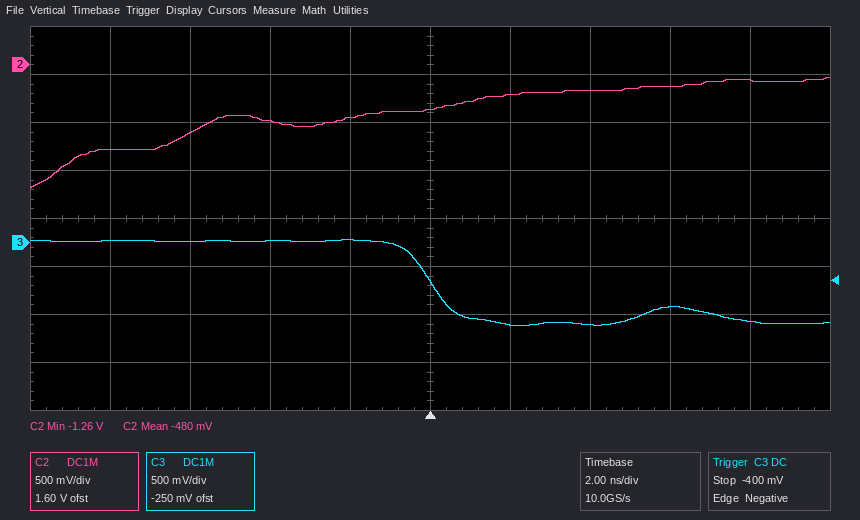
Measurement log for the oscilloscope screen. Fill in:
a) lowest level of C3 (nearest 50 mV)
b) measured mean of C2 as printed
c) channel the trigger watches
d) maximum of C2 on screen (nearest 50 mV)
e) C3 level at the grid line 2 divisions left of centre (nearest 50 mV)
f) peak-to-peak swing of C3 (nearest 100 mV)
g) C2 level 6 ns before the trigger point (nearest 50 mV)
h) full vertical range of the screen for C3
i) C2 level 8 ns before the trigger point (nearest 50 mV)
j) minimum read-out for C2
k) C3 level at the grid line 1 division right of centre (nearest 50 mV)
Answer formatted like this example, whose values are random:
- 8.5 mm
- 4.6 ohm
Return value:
- -850 mV
- -480 mV
- C3
- -150 mV
- 0 mV
- 900 mV
- -700 mV
- 4 V
- -900 mV
- -1.26 V
- -850 mV
